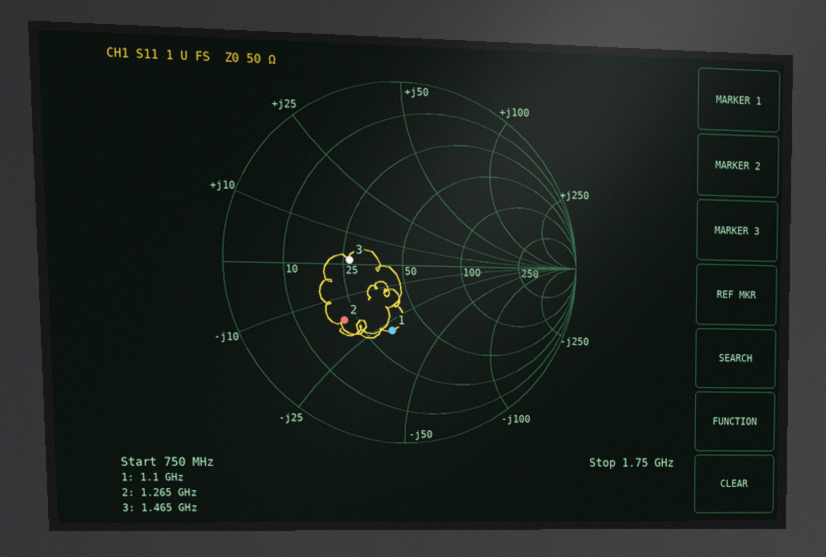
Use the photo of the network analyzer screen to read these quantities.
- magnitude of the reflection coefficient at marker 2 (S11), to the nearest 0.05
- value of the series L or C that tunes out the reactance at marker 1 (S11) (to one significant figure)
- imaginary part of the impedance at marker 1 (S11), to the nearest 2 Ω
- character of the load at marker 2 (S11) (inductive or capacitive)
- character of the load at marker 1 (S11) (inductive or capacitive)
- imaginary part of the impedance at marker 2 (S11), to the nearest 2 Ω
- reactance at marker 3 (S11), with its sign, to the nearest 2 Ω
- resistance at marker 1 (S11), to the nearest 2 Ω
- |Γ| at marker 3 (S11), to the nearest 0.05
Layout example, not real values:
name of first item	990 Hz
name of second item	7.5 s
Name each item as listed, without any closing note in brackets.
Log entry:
magnitude of the reflection coefficient at marker 2 (S11), to the nearest 0.05	0.45
value of the series L or C that tunes out the reactance at marker 1 (S11)	4 nH
imaginary part of the impedance at marker 1 (S11), to the nearest 2 Ω	-28 Ω
character of the load at marker 2 (S11)	capacitive
character of the load at marker 1 (S11)	capacitive
imaginary part of the impedance at marker 2 (S11), to the nearest 2 Ω	-16 Ω
reactance at marker 3 (S11), with its sign, to the nearest 2 Ω	+2 Ω
resistance at marker 1 (S11), to the nearest 2 Ω	34 Ω
|Γ| at marker 3 (S11), to the nearest 0.05	0.30
